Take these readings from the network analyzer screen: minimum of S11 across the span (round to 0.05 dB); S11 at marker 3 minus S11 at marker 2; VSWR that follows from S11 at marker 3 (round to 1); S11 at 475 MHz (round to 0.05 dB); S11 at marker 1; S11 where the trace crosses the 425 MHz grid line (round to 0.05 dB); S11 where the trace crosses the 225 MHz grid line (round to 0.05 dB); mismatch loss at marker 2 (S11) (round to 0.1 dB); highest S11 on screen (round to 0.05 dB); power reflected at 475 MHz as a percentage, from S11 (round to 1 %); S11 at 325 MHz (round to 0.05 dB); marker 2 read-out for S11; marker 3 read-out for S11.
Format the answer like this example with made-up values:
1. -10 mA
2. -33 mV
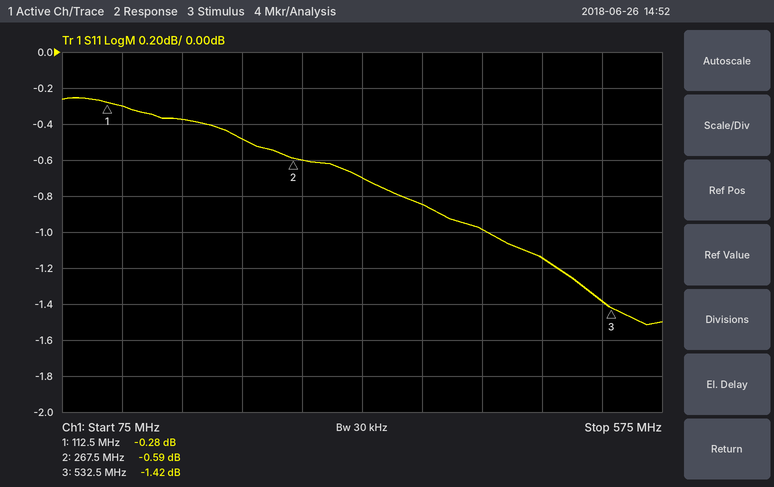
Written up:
1. -1.50 dB
2. -0.83 dB
3. 12
4. -1.15 dB
5. -0.28 dB
6. -1.00 dB
7. -0.50 dB
8. 9.0 dB
9. -0.25 dB
10. 77 %
11. -0.70 dB
12. -0.59 dB
13. -1.42 dB
